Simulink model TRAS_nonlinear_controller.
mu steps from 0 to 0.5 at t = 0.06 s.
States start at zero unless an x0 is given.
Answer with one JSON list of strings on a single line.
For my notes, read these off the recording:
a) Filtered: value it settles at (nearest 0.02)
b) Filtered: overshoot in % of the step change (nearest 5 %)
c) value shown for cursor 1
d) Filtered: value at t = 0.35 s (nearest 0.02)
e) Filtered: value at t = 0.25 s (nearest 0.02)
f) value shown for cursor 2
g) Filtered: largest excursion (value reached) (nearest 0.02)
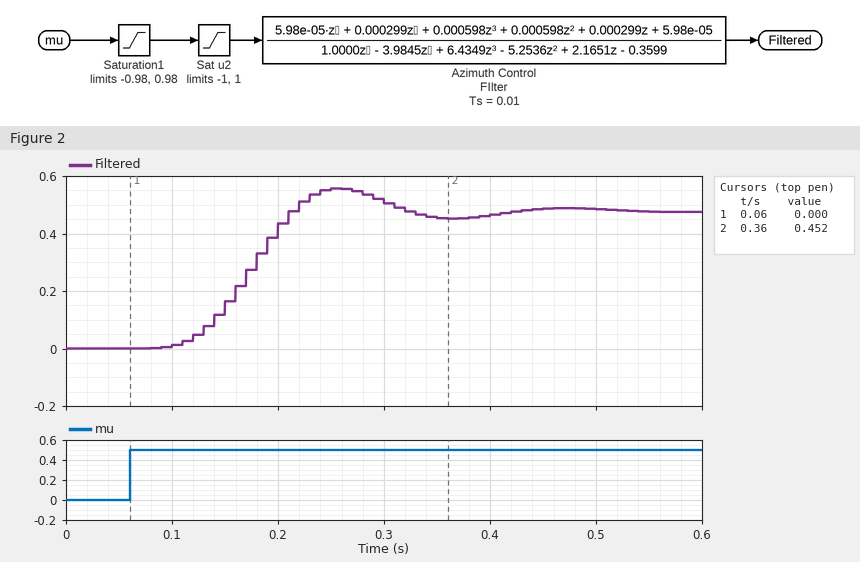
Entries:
["0.48", "15 %", "0.000", "0.46", "0.56", "0.452", "0.56"]
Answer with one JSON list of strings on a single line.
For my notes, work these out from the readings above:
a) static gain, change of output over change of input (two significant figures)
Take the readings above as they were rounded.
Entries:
["0.96"]
